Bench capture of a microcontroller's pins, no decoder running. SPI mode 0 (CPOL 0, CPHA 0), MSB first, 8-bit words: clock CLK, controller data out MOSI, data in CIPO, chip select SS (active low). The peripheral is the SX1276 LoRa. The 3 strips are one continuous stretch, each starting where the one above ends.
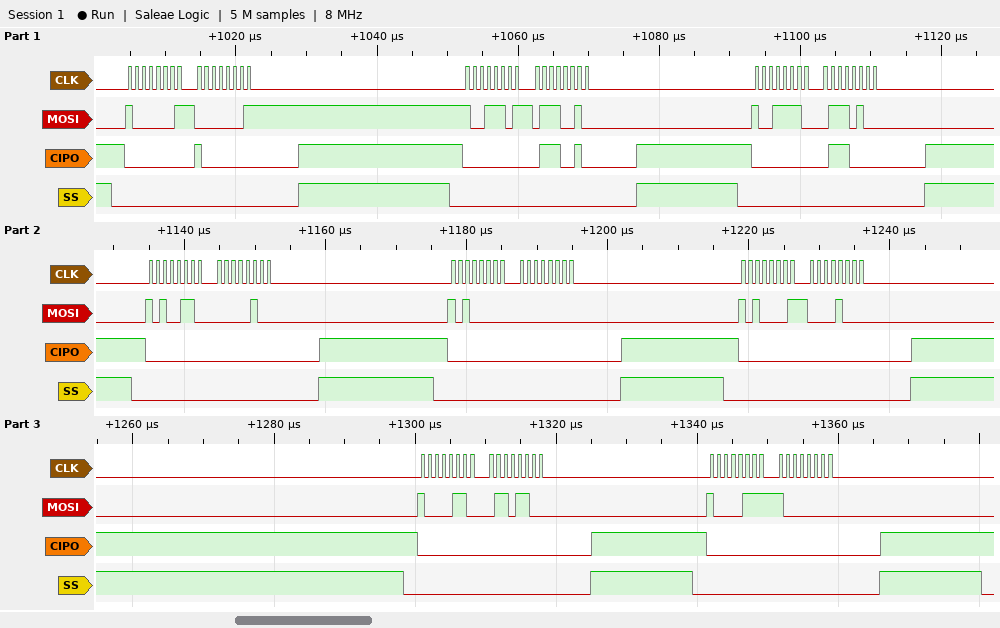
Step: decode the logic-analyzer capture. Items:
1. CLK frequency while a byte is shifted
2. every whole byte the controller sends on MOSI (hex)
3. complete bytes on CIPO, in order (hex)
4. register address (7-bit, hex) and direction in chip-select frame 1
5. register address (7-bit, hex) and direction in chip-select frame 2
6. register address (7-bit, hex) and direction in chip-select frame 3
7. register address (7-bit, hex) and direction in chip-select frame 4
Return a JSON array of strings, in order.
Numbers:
["1 MHz", "81 01 9D 72 9E 74 A6 04 A0 00 A1 08 86 6C 87 80", "00 80 00 72 00 70 00 00 00 00 00 00 00 00 00 00", "0x01 write", "0x1D write", "0x1E write", "0x26 write"]
